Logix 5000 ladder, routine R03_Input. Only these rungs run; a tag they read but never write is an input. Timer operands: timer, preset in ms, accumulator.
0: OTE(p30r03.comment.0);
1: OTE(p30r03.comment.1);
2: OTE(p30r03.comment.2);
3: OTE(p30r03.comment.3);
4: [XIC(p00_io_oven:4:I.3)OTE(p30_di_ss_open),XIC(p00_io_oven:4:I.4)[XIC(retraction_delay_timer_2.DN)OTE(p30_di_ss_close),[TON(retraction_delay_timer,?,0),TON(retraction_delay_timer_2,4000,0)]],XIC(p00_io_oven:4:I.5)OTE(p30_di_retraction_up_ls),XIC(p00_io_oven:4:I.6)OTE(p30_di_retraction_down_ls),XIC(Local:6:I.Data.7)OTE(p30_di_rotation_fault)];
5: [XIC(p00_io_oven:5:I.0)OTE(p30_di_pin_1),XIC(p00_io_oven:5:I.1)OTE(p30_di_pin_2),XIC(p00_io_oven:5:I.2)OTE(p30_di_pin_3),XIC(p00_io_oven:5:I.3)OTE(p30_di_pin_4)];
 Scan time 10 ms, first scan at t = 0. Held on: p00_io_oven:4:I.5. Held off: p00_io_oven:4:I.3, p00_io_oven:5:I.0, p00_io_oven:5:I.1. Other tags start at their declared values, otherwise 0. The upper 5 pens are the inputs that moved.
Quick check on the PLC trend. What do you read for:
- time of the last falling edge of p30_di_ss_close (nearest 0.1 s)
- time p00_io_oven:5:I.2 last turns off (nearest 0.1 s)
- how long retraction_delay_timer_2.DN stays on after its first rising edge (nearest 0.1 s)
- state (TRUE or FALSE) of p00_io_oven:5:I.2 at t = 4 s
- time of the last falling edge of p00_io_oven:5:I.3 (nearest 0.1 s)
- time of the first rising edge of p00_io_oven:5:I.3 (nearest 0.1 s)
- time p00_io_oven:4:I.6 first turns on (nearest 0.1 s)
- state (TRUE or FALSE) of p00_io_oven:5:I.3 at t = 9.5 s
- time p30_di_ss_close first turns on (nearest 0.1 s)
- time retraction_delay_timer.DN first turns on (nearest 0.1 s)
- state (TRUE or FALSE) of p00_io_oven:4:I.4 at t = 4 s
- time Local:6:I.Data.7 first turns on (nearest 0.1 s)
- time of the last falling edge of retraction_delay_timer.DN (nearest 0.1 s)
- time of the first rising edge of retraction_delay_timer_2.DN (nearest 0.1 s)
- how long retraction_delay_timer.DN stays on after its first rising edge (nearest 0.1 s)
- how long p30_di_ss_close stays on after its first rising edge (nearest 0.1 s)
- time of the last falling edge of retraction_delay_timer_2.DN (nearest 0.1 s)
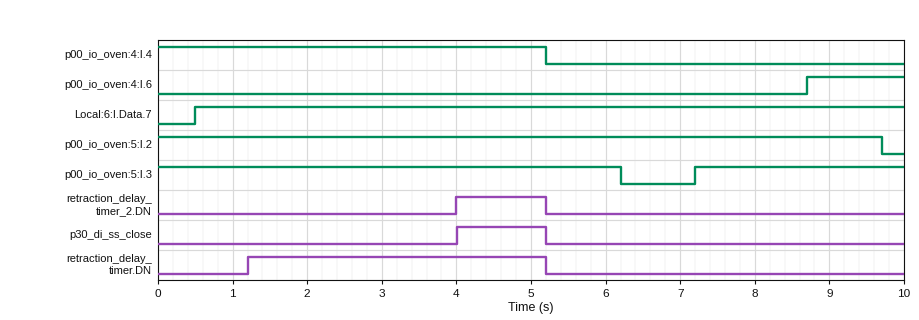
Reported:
5.2 s
9.7 s
1.2 s
TRUE
6.2 s
7.2 s
8.7 s
TRUE
4.0 s
1.2 s
TRUE
0.5 s
5.2 s
4.0 s
4.0 s
1.2 s
5.2 s
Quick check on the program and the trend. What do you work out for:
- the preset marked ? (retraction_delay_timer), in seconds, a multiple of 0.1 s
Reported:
1.2 s
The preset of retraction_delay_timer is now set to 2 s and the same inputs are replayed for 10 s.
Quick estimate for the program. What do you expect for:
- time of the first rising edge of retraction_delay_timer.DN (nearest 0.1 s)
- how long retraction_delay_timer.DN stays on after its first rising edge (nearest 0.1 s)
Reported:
2.0 s
3.2 s
